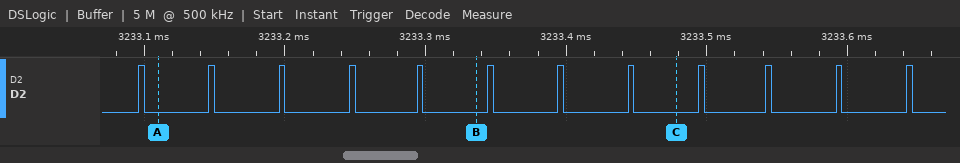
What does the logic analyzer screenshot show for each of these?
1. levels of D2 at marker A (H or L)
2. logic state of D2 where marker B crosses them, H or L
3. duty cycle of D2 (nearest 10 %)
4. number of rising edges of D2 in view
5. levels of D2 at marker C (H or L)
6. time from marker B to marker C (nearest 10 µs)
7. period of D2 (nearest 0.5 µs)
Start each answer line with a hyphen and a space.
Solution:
- D2=L
- D2=L
- 10 %
- 12
- D2=L
- 140 µs
- 49.5 µs
